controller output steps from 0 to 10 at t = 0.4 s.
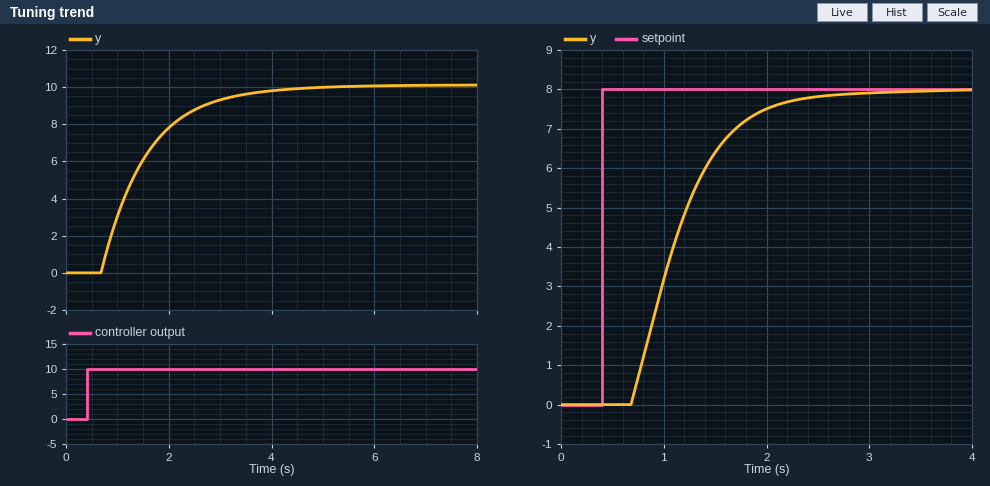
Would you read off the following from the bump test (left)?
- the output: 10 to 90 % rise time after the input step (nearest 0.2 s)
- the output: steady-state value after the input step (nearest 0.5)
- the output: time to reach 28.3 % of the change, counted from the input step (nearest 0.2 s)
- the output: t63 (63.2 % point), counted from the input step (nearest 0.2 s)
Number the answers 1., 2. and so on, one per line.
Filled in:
1. 2.0 s
2. 10.0
3. 0.6 s
4. 1.2 s
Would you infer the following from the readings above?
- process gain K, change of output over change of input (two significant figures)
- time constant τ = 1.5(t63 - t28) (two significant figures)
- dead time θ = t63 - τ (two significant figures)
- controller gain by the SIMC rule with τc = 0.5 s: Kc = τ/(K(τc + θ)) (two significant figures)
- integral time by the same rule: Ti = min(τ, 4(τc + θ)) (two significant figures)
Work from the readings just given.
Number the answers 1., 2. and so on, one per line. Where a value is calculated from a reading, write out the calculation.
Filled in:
1. (10 - 0) / 10 = 1.0
2. 1.5 × (1.2 - 0.6) = 0.90 s
3. 1.2 - 0.9 = 0.30 s
4. 0.9 / (1 × (0.5 + 0.3)) = 1.1
5. min(0.9, 4 × (0.5 + 0.3)) = 0.90 s
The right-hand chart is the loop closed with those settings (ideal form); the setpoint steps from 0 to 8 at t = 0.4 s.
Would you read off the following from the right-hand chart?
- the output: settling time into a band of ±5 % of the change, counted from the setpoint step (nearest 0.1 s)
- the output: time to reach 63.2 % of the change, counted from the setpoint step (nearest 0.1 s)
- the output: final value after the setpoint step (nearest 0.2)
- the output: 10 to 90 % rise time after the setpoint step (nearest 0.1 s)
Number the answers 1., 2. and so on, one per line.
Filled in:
1. 1.7 s
2. 0.8 s
3. 8.0
4. 1.0 s
